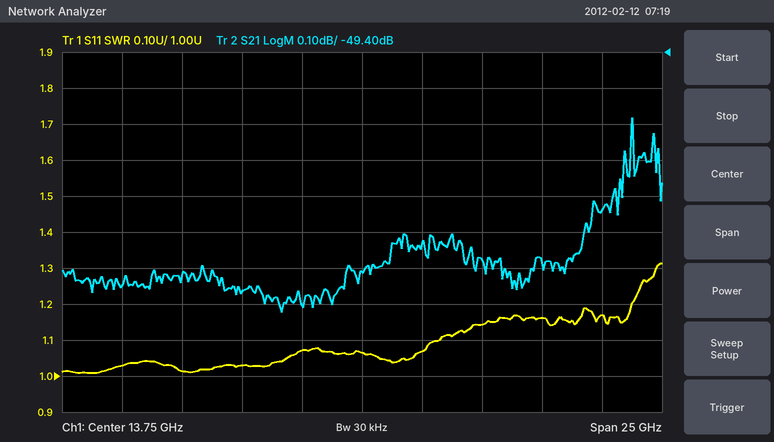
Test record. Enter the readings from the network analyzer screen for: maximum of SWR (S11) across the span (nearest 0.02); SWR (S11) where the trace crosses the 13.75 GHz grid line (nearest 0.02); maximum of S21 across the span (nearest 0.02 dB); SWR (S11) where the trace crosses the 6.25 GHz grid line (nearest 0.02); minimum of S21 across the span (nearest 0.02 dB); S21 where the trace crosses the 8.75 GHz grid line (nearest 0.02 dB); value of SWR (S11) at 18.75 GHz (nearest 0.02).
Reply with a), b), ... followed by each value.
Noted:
a) 1.32
b) 1.06
c) -49.58 dB
d) 1.02
e) -50.12 dB
f) -50.06 dB
g) 1.14
